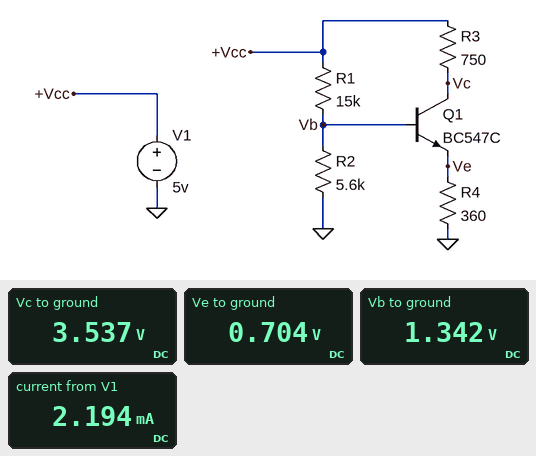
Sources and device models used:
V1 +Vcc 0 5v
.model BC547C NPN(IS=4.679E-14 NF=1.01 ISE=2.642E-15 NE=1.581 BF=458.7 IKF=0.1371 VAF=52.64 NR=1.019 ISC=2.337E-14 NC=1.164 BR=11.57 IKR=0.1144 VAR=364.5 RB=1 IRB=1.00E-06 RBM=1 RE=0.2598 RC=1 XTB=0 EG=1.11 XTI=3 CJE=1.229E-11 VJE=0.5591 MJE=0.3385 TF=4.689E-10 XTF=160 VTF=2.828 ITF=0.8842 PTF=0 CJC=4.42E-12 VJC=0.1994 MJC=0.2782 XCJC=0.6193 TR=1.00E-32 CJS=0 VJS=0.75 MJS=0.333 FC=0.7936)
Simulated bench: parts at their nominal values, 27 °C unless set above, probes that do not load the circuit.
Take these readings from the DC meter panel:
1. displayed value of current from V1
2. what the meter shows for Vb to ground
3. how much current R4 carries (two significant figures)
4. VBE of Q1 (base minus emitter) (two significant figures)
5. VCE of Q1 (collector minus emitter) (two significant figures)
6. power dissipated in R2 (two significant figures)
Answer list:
2.194 mA
1.342 V
2.0 mA
640 mV
2.8 V
320 µW
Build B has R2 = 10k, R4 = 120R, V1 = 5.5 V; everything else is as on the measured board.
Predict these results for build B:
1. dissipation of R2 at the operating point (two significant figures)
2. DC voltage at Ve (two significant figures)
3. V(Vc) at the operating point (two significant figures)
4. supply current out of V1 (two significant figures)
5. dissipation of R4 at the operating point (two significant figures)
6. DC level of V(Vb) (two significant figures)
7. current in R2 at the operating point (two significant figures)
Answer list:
210 µW
760 mV
820 mV
6.5 mA
4.9 mW
1.4 V
140 µA
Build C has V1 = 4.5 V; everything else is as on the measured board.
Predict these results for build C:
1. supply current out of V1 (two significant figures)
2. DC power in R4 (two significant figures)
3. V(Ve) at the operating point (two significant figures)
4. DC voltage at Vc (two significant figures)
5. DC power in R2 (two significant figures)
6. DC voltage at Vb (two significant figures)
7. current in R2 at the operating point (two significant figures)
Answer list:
1.8 mA
920 µW
580 mV
3.3 V
260 µW
1.2 V
220 µA
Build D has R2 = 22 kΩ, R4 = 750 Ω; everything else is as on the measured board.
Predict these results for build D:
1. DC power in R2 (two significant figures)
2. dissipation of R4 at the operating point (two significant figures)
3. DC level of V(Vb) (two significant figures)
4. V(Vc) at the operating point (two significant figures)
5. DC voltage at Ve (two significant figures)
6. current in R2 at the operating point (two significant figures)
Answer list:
390 µW
6.8 mW
2.9 V
2.7 V
2.3 V
130 µA
